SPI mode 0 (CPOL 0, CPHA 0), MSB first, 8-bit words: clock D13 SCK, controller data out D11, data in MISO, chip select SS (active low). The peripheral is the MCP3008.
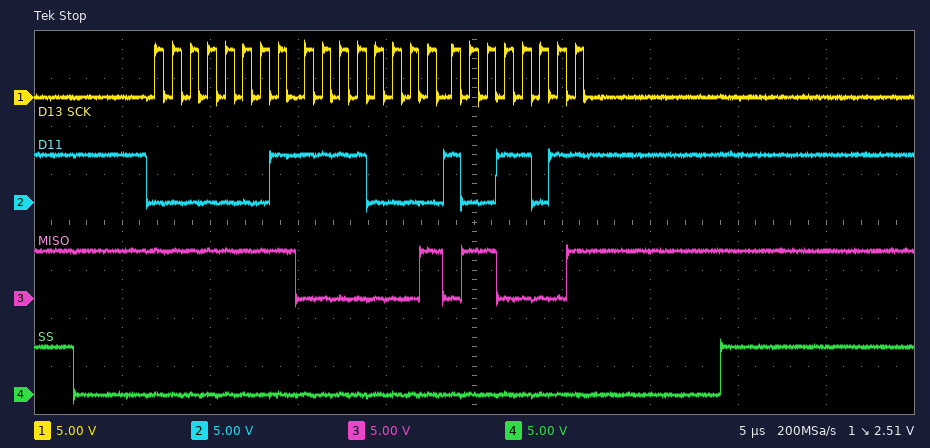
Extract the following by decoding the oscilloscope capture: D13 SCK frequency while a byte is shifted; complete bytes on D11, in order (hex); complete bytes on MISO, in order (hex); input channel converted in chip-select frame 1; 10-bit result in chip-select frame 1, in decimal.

1 MHz
01 F0 9B
FF 01 61
7
353
